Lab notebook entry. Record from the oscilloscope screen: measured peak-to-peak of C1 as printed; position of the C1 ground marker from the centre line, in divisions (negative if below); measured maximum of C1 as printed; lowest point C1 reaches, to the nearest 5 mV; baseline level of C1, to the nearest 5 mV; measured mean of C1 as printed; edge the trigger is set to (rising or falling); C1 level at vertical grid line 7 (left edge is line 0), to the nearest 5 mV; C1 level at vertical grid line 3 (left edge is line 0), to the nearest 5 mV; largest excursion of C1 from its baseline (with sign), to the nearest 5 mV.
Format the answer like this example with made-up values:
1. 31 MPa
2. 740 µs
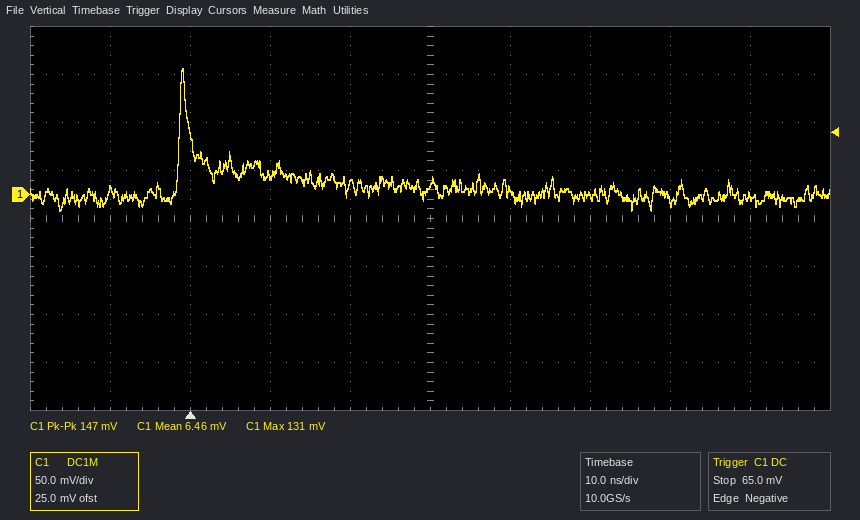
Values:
1. 147 mV
2. +0.5 div
3. 131 mV
4. -15 mV
5. 0 mV
6. 6.46 mV
7. falling
8. 0 mV
9. 20 mV
10. +130 mV
